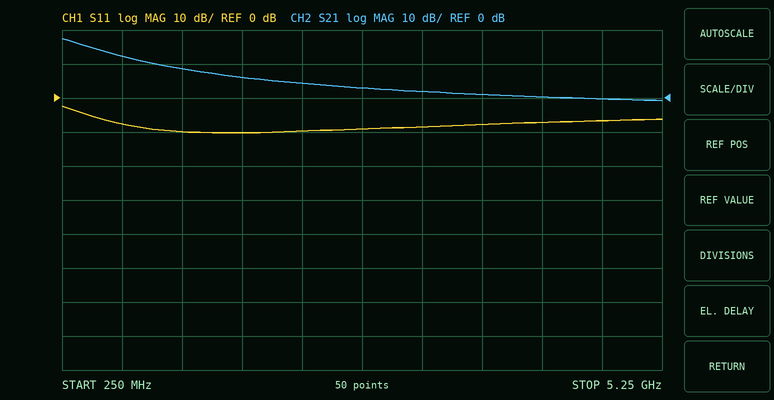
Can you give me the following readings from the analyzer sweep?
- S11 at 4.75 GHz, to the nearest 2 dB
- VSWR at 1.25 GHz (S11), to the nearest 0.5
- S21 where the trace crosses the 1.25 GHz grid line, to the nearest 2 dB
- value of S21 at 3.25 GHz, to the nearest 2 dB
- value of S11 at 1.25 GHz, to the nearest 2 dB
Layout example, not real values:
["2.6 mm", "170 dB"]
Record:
["-6 dB", "2.0", "8 dB", "2 dB", "-10 dB"]
